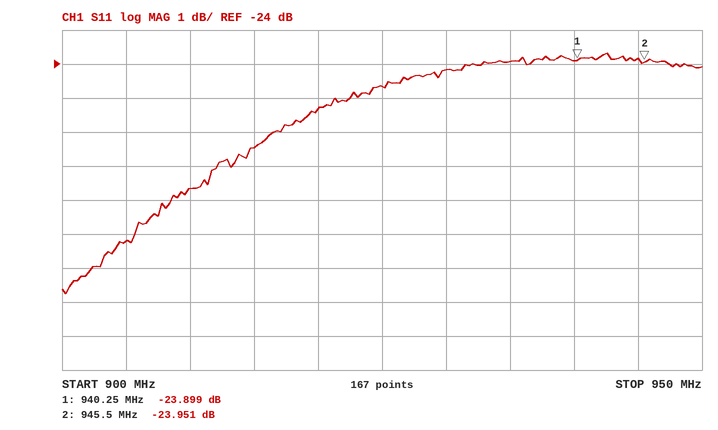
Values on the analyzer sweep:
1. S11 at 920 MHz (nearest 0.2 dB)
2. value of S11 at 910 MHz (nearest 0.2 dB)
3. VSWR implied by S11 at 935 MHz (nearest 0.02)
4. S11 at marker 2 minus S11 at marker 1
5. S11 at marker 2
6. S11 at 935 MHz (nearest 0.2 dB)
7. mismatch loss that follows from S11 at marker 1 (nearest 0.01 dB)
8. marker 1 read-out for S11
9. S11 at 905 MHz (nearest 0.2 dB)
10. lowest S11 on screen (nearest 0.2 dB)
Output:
-25.4 dB
-27.6 dB
1.14
-0.052 dB
-23.951 dB
-24.0 dB
0.02 dB
-23.899 dB
-29.2 dB
-30.8 dB
